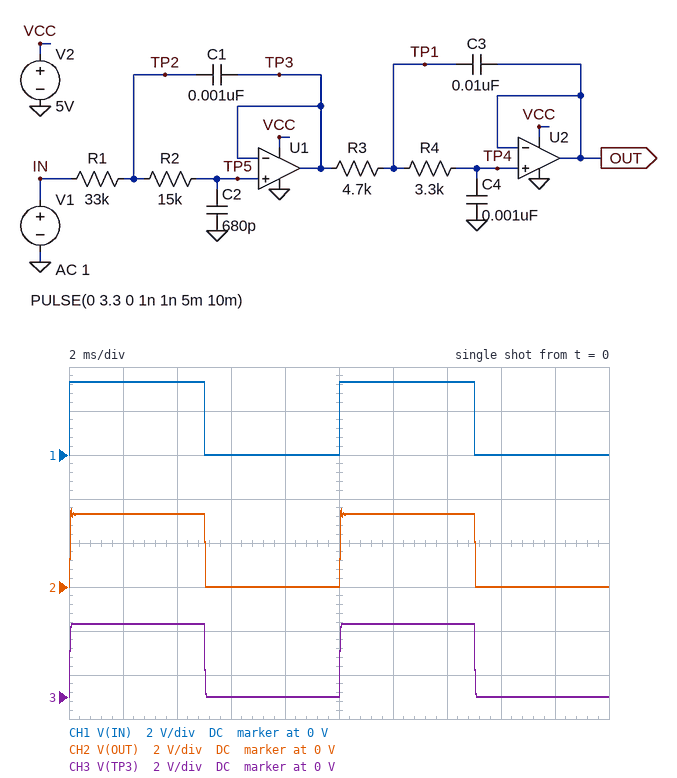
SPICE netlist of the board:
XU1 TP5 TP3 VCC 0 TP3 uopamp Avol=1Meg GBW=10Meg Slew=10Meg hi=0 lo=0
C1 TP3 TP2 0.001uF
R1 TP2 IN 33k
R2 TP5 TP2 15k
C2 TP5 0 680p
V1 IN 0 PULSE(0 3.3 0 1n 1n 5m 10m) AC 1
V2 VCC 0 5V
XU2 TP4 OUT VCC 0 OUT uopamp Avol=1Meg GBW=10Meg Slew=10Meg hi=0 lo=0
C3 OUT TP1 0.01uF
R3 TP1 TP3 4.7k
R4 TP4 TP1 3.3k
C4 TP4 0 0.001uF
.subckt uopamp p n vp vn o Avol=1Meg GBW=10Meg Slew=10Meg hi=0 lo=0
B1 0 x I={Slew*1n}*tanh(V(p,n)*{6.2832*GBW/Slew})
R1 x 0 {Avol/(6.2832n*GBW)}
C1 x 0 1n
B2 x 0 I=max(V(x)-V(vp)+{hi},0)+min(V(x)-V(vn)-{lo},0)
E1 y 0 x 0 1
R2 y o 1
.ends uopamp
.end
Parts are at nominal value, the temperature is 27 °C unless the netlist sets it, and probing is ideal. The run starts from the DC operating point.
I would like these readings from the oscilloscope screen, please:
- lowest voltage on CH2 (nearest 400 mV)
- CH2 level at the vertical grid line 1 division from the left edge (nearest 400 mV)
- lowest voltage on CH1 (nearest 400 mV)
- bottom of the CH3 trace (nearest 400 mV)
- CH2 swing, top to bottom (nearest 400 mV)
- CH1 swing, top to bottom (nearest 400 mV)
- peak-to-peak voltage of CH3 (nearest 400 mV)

0 V
3.2 V
0 V
0 V
3.6 V
3.2 V
3.2 V
